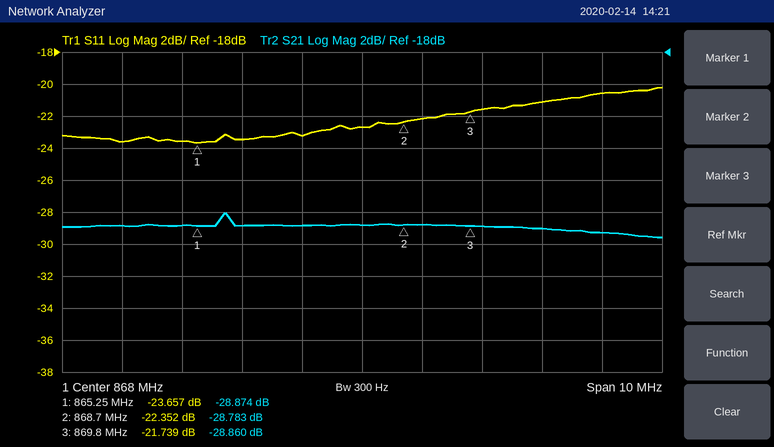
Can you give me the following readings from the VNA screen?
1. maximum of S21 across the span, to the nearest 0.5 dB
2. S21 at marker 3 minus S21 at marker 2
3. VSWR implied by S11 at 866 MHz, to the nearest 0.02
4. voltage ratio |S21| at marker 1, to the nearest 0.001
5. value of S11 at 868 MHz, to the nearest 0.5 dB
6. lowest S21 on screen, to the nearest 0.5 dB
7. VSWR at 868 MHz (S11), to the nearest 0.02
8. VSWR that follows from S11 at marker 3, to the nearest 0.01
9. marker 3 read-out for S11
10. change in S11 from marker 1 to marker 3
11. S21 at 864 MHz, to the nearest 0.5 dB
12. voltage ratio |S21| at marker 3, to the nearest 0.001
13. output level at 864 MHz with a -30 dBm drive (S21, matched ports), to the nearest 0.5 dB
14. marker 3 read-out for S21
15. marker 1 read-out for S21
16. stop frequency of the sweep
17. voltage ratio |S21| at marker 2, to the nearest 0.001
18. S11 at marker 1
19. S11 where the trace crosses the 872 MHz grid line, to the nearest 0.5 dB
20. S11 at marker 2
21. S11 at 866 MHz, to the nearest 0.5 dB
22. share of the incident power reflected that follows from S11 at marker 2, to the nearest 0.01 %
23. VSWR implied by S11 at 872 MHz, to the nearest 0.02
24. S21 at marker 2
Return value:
-28.0 dB
-0.077 dB
1.14
0.036
-22.5 dB
-29.5 dB
1.16
1.18
-21.739 dB
1.918 dB
-29.0 dB
0.036
-59.0 dBm
-28.860 dB
-28.874 dB
873 MHz
0.036
-23.657 dB
-20.5 dB
-22.352 dB
-23.5 dB
0.58 %
1.20
-28.783 dB
